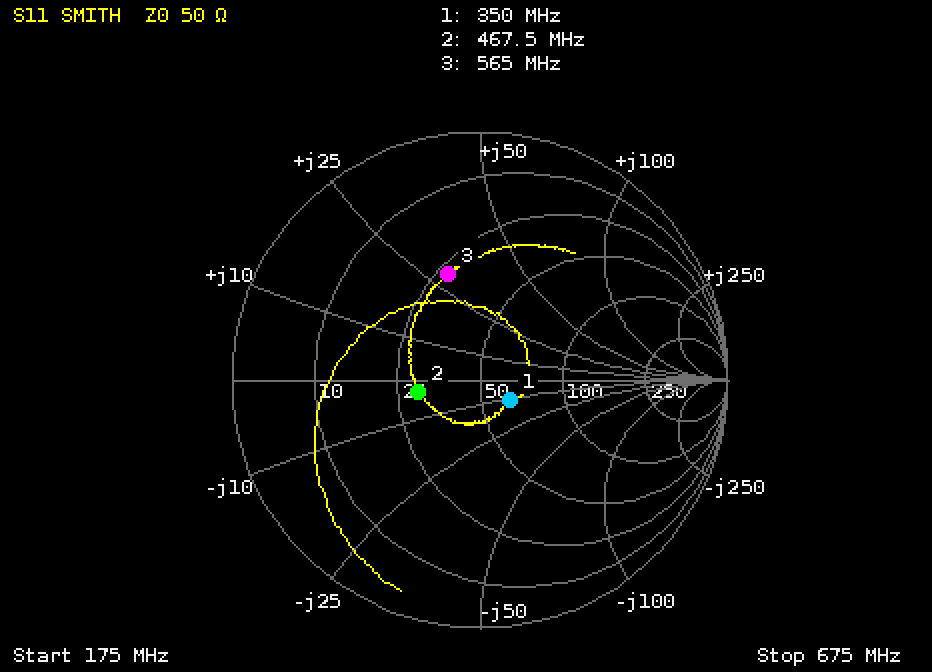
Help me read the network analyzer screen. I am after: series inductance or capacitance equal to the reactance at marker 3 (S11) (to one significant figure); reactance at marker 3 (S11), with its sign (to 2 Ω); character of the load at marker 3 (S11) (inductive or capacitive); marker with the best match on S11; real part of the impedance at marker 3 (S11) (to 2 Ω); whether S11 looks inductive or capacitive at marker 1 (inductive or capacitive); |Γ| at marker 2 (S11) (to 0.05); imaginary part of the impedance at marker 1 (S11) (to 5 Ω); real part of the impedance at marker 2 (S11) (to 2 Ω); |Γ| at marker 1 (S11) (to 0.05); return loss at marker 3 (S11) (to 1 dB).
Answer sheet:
8 nH
+30 Ω
inductive
marker 1
28 Ω
capacitive
0.25
-10 Ω
30 Ω
0.15
7 dB
